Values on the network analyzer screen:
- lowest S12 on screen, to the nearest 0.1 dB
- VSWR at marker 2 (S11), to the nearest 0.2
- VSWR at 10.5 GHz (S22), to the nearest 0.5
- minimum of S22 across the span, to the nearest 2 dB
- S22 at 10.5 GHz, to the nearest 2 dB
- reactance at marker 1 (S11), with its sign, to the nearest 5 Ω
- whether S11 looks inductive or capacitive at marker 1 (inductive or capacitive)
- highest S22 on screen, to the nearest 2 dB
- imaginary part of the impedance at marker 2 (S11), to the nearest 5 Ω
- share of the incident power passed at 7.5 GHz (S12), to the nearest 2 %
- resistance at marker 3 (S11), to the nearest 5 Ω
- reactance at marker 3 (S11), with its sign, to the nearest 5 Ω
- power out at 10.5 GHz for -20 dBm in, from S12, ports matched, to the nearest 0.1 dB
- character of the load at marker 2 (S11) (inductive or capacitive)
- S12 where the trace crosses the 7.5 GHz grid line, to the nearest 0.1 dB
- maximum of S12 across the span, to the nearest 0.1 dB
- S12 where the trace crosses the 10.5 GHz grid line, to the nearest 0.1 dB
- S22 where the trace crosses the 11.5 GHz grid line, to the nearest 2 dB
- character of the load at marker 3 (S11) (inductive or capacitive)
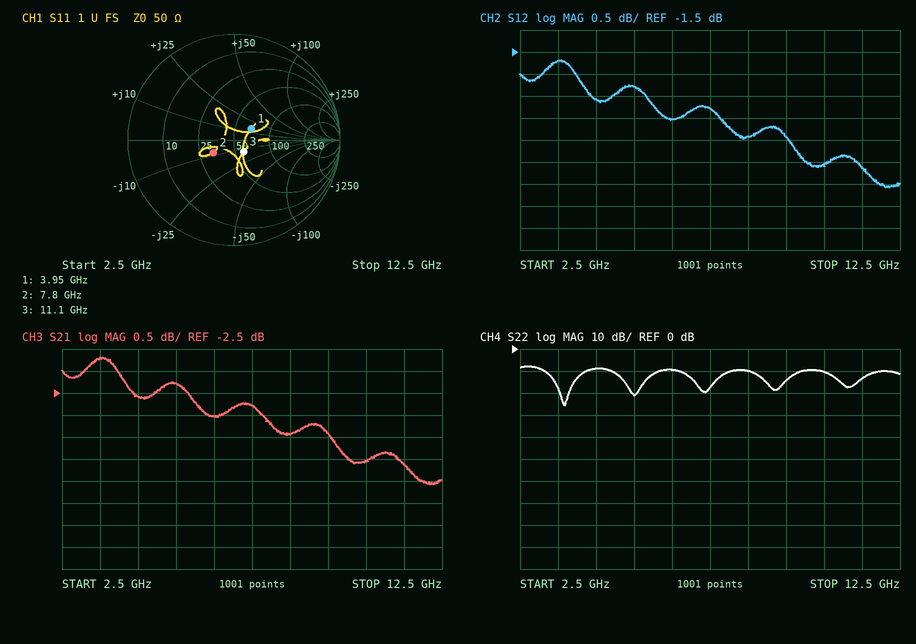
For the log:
-4.6 dB
1.6
2.0
-26 dB
-10 dB
+15 Ω
inductive
-8 dB
-10 Ω
52 %
60 Ω
-15 Ω
-24.1 dBm
capacitive
-2.8 dB
-1.7 dB
-4.1 dB
-14 dB
capacitive
